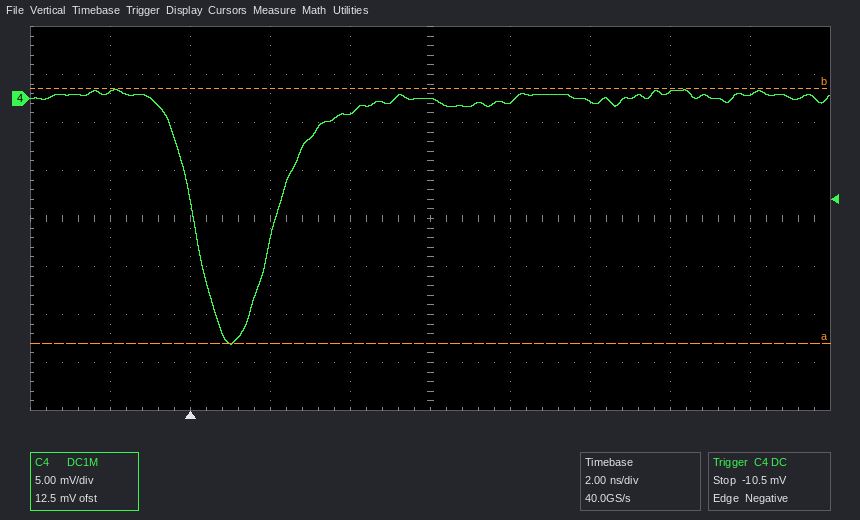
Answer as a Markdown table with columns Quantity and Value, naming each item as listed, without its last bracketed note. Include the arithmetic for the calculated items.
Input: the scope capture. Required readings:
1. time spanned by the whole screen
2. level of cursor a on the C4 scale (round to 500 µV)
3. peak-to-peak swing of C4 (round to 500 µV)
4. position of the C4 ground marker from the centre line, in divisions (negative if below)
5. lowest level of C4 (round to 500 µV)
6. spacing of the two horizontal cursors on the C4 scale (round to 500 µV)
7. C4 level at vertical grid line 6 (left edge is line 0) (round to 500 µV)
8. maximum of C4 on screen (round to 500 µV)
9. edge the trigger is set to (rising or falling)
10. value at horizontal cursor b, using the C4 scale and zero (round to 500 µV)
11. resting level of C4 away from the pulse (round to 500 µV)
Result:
| Quantity | Value |
|---|---|
| time spanned by the whole screen | 20 ns |
| level of cursor a on the C4 scale | -25.5 mV |
| peak-to-peak swing of C4 | 1.0 mV − (-25.5 mV) = 26.5 mV |
| position of the C4 ground marker from the centre line, in divisions | +2.5 div |
| lowest level of C4 | -25.5 mV |
| spacing of the two horizontal cursors on the C4 scale | 26.5 mV |
| C4 level at vertical grid line 6 (left edge is line 0) | -500 µV |
| maximum of C4 on screen | 1.0 mV |
| edge the trigger is set to | falling |
| value at horizontal cursor b, using the C4 scale and zero | 1.0 mV |
| resting level of C4 away from the pulse | 0.0 mV |
